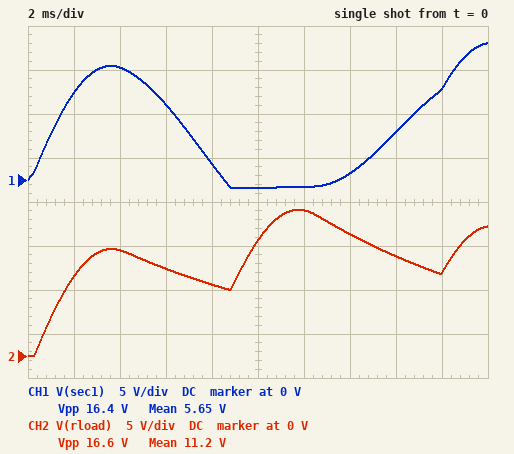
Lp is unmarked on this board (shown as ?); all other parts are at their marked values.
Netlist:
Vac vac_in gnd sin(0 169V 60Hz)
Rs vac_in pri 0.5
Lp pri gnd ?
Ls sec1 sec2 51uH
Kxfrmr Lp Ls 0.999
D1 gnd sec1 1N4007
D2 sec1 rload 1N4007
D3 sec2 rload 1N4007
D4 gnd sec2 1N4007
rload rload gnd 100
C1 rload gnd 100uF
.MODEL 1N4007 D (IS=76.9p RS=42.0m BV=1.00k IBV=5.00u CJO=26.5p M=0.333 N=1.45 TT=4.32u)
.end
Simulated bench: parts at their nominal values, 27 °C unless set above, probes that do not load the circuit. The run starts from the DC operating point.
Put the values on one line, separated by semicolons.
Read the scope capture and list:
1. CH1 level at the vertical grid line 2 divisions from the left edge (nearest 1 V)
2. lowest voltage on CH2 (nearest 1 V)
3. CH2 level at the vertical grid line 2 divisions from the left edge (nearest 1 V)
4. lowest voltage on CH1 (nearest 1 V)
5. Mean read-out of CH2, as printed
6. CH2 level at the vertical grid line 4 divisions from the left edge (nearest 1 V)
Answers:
13 V; 0 V; 12 V; -1 V; 11.2 V; 8 V
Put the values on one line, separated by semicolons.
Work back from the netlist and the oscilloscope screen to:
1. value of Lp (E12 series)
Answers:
4.7 mH
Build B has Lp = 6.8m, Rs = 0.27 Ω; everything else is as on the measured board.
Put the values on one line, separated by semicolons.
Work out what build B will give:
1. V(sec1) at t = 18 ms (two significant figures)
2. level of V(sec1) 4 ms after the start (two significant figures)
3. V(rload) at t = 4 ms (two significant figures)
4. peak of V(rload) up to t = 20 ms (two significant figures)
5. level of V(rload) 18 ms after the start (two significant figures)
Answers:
7.8 V; 12 V; 12 V; 14 V; 8.1 V
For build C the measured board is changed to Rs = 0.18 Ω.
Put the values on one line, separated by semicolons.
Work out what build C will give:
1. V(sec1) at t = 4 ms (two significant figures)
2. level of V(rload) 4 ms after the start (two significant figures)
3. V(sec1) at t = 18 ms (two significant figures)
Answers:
15 V; 14 V; 9.5 V
